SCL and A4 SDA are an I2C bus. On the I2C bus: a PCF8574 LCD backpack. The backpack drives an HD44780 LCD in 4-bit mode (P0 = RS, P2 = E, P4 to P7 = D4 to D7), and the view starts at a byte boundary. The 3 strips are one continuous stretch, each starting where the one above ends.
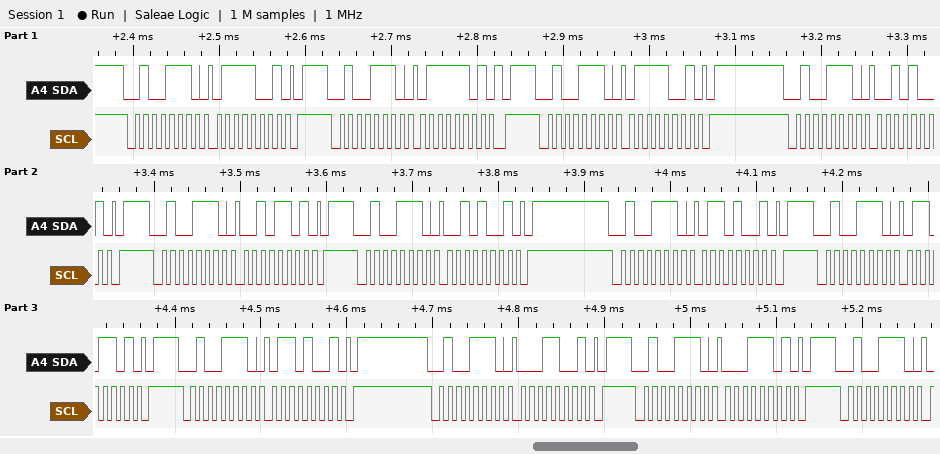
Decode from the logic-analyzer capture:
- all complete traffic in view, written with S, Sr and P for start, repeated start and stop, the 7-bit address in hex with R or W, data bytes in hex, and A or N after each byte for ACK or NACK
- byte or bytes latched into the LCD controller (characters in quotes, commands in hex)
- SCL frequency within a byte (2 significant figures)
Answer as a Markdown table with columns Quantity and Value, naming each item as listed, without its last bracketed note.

| Quantity | Value |
|---|---|
| all complete traffic in view, written with S, Sr and P for start, repeated start and stop, the 7-bit address in hex with R or W, data bytes in hex, and A or N after each byte for ACK or NACK | S 27W A 79 A P S 27W A 7D A P S 27W A 79 A P S 27W A 29 A P S 27W A 2D A P S 27W A 29 A P S 27W A 69 A P S 27W A 6D A P S 27W A 69 A P S 27W A 19 A P S 27W A 1D A P S 27W A |
| byte or bytes latched into the LCD controller | 'r' |
| SCL frequency within a byte | 100 kHz |
